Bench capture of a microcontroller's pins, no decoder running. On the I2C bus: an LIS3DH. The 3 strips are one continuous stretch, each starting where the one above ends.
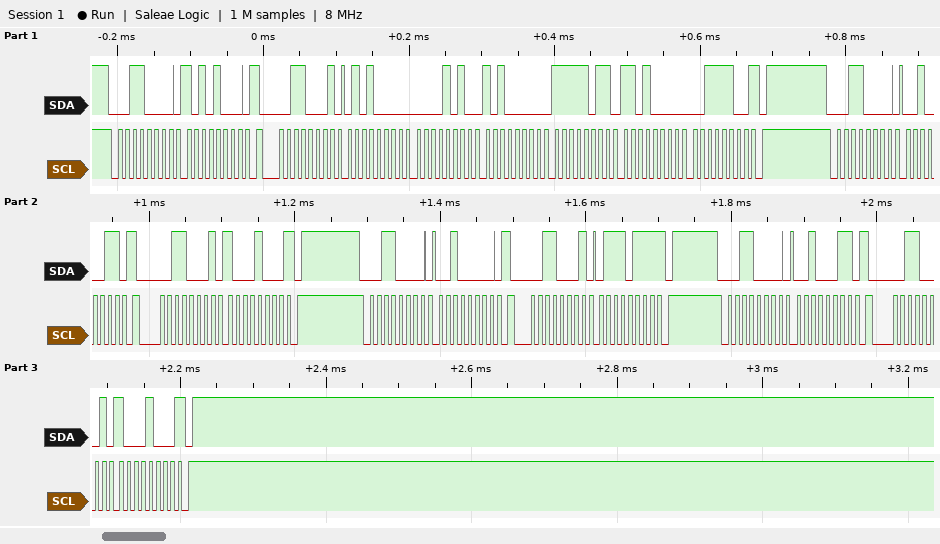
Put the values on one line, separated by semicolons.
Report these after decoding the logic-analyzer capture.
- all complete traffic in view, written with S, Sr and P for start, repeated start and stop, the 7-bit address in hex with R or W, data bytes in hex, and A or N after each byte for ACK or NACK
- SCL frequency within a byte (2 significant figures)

S 18W A A8 A Sr 18R A 50 A 0A A A0 A FB A D0 A 3C N P S 18W A 23 A Sr 18R A 88 N P S 18W A 20 A Sr 18R A 77 N P S 18W A 23 A Sr 18R A 88 N P; 100 kHz
